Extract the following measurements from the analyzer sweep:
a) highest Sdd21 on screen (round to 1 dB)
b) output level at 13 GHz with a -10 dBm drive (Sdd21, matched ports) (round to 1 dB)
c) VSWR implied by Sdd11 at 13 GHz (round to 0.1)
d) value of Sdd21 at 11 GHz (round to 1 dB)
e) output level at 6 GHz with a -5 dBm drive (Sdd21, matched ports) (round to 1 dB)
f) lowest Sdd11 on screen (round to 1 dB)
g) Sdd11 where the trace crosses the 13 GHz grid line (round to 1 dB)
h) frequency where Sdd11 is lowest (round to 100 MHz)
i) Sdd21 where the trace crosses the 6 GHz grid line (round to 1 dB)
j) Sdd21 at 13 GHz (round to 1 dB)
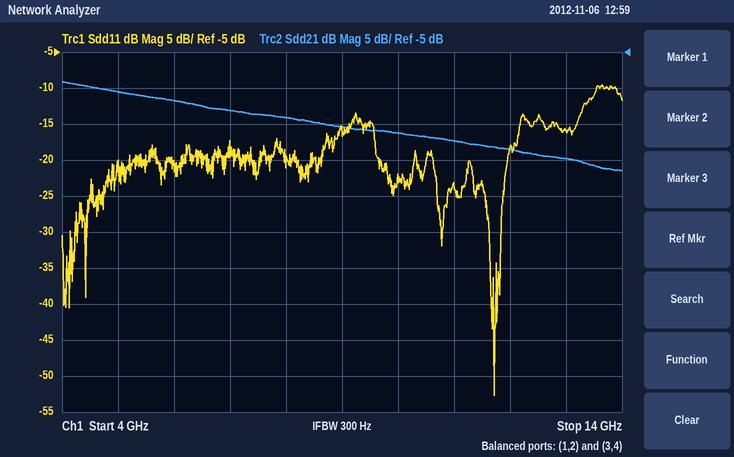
-9 dB
-30 dBm
1.4
-17 dB
-17 dBm
-53 dB
-16 dB
11.7 GHz
-12 dB
-20 dB
